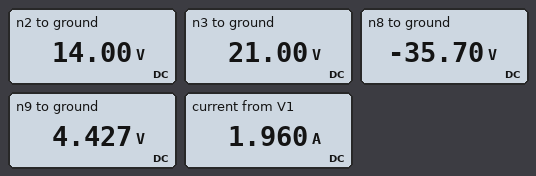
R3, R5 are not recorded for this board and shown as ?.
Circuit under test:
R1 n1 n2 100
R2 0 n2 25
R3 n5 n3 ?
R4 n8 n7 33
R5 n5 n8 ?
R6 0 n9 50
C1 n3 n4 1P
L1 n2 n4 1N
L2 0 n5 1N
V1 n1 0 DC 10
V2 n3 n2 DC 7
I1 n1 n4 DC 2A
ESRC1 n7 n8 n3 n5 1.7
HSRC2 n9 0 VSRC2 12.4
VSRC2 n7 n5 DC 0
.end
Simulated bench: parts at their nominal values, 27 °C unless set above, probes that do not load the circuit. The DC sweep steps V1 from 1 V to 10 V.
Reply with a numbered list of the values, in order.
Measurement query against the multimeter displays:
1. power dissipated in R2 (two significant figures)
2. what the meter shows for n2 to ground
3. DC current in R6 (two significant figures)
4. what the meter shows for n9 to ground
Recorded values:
1. 7.8 W
2. 14.00 V
3. 89 mA
4. 4.427 V
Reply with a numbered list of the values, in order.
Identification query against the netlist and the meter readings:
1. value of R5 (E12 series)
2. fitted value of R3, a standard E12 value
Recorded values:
1. 100 Ω
2. 15 Ω
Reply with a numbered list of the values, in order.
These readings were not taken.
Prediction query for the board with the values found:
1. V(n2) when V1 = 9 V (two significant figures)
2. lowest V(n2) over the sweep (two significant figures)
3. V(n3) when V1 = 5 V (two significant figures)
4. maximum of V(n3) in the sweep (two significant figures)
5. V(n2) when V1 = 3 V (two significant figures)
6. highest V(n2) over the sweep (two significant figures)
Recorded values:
1. 14 V
2. 13 V
3. 21 V
4. 21 V
5. 13 V
6. 14 V
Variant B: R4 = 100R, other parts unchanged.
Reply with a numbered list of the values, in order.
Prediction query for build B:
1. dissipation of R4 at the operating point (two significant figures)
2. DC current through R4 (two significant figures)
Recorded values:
1. 13 W
2. 360 mA
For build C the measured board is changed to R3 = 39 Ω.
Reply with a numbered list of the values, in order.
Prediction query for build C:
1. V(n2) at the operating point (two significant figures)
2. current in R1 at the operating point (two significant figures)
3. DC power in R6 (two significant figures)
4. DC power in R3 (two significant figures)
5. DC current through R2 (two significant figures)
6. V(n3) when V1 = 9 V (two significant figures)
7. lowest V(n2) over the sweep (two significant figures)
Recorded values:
1. 25 V
2. 150 mA
3. 930 mW
4. 27 W
5. 1.0 A
6. 32 V
7. 24 V
